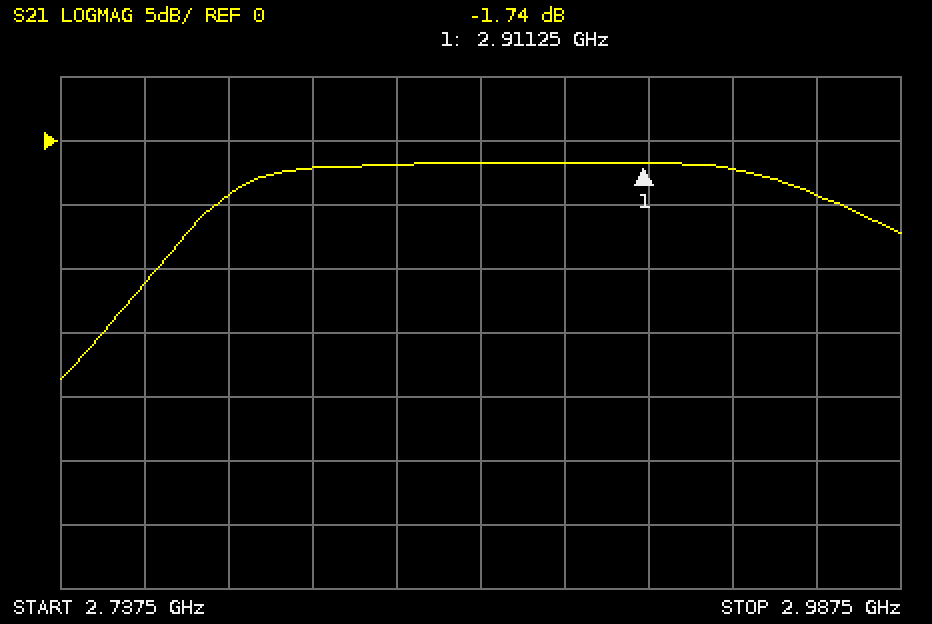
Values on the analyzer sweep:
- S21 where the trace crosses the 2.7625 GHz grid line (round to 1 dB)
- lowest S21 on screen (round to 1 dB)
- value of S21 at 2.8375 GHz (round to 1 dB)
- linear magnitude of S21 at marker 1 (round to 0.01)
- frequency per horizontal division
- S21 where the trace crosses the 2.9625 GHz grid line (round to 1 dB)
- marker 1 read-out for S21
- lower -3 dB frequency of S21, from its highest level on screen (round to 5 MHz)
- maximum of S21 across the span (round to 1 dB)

-11 dB
-19 dB
-2 dB
0.82
25 MHz
-4 dB
-1.74 dB
2.785 GHz
-2 dB
